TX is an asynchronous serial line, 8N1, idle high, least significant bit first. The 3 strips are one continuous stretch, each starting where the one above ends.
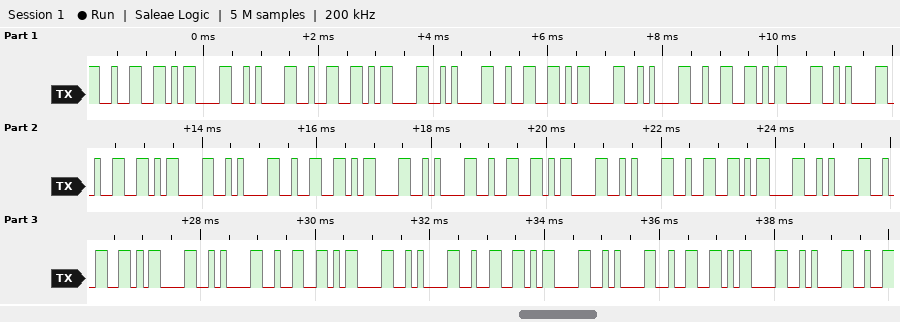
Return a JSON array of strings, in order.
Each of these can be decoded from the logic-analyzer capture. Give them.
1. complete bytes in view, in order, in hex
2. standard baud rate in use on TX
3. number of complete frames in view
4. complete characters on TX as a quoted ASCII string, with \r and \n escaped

["32 0D 0A 32 0D 0A 32 0D 0A 32 0D 0A 32 0D 0A 32 0D 0A 32 0D 0A 32 0D 0A 32 0D 0A 32 0D 0A 32 0D 0A 32 0D 0A", "9600 baud", "36", "\"2\\r\\n2\\r\\n2\\r\\n2\\r\\n2\\r\\n2\\r\\n2\\r\\n2\\r\\n2\\r\\n2\\r\\n2\\r\\n2\\r\\n\""]
